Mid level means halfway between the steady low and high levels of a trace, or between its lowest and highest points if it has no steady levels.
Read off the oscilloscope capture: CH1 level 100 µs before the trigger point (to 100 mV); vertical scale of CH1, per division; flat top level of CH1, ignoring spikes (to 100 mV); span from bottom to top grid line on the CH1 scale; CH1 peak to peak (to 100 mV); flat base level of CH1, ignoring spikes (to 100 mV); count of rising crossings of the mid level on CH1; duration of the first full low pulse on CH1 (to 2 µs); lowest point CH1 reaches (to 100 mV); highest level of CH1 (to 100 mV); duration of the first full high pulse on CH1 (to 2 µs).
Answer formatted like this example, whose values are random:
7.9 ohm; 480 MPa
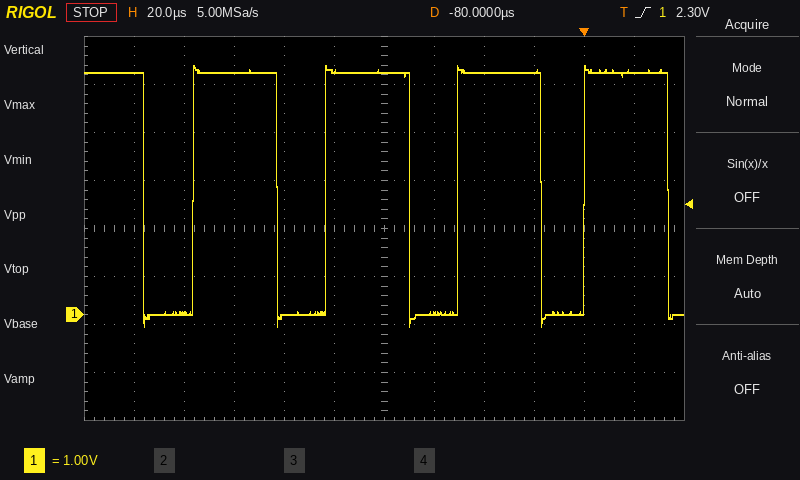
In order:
5.1 V; 1 V; 5.0 V; 8 V; 5.4 V; 0.0 V; 4; 20 µs; -200 mV; 5.2 V; 34 µs
